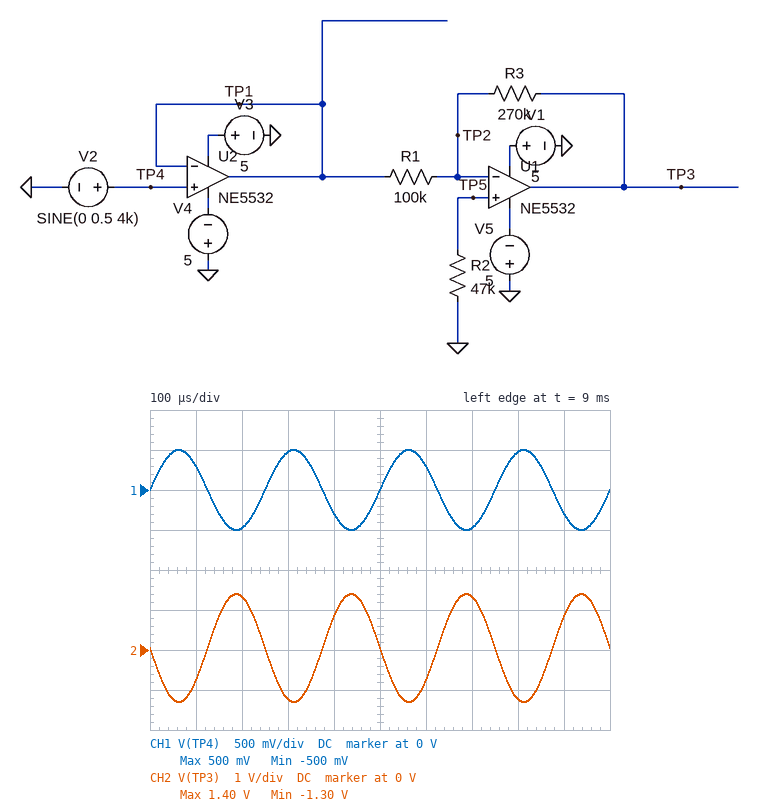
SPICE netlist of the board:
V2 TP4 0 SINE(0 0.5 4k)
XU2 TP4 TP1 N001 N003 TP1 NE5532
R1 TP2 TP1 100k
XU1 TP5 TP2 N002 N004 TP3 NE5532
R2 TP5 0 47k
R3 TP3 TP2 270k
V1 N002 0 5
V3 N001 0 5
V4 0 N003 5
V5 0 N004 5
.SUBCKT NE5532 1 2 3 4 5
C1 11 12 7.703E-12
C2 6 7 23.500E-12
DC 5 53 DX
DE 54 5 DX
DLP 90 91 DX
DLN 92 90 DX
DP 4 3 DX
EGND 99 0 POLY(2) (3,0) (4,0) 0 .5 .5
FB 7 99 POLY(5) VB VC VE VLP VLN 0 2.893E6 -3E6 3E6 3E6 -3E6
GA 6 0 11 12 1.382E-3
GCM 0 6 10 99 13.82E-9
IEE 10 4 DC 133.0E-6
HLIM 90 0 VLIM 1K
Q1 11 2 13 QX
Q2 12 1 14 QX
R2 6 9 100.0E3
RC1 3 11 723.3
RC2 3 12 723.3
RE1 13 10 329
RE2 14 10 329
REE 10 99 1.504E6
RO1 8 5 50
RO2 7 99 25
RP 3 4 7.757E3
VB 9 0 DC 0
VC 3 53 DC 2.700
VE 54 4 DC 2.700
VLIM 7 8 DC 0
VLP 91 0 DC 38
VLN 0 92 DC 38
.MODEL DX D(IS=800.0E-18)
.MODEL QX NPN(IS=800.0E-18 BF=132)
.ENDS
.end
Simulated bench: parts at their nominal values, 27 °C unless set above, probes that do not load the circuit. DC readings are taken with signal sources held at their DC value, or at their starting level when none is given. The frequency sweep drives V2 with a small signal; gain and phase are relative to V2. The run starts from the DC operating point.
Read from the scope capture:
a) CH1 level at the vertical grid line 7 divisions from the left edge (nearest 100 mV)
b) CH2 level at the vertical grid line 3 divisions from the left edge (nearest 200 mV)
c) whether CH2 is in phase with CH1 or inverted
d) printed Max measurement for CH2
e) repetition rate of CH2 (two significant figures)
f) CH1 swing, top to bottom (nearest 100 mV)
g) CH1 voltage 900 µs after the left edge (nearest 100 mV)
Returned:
-500 mV
-1.2 V
inverted
1.40 V
4.0 kHz
1.0 V
-300 mV
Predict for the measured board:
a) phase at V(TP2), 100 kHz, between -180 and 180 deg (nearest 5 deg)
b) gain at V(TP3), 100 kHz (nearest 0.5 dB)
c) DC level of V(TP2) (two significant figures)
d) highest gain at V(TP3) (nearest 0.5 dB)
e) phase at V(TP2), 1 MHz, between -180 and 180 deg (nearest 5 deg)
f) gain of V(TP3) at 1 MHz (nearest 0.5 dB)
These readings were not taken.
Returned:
85 deg
8.5 dB
-23 mV
8.5 dB
55 deg
7.5 dB
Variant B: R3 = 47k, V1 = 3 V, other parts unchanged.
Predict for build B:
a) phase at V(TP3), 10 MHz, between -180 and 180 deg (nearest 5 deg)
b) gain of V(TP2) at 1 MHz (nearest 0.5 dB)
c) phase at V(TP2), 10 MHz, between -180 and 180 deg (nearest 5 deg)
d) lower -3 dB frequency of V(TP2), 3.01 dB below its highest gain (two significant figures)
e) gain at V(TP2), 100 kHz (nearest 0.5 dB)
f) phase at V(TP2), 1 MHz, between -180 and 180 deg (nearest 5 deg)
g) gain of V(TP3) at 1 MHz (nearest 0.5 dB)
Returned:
0 deg
-24.0 dB
-55 deg
4.0 MHz
-44.0 dB
75 deg
-6.5 dB
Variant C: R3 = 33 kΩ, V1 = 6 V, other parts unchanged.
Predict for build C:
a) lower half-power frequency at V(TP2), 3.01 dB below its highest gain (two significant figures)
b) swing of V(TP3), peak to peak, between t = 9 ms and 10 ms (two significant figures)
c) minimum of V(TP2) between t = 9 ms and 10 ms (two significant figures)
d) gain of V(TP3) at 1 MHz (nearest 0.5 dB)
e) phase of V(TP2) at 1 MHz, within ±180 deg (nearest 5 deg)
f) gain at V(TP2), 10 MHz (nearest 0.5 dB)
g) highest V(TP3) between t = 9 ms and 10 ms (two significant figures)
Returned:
4.3 MHz
330 mV
-23 mV
-9.5 dB
75 deg
-12.0 dB
150 mV
